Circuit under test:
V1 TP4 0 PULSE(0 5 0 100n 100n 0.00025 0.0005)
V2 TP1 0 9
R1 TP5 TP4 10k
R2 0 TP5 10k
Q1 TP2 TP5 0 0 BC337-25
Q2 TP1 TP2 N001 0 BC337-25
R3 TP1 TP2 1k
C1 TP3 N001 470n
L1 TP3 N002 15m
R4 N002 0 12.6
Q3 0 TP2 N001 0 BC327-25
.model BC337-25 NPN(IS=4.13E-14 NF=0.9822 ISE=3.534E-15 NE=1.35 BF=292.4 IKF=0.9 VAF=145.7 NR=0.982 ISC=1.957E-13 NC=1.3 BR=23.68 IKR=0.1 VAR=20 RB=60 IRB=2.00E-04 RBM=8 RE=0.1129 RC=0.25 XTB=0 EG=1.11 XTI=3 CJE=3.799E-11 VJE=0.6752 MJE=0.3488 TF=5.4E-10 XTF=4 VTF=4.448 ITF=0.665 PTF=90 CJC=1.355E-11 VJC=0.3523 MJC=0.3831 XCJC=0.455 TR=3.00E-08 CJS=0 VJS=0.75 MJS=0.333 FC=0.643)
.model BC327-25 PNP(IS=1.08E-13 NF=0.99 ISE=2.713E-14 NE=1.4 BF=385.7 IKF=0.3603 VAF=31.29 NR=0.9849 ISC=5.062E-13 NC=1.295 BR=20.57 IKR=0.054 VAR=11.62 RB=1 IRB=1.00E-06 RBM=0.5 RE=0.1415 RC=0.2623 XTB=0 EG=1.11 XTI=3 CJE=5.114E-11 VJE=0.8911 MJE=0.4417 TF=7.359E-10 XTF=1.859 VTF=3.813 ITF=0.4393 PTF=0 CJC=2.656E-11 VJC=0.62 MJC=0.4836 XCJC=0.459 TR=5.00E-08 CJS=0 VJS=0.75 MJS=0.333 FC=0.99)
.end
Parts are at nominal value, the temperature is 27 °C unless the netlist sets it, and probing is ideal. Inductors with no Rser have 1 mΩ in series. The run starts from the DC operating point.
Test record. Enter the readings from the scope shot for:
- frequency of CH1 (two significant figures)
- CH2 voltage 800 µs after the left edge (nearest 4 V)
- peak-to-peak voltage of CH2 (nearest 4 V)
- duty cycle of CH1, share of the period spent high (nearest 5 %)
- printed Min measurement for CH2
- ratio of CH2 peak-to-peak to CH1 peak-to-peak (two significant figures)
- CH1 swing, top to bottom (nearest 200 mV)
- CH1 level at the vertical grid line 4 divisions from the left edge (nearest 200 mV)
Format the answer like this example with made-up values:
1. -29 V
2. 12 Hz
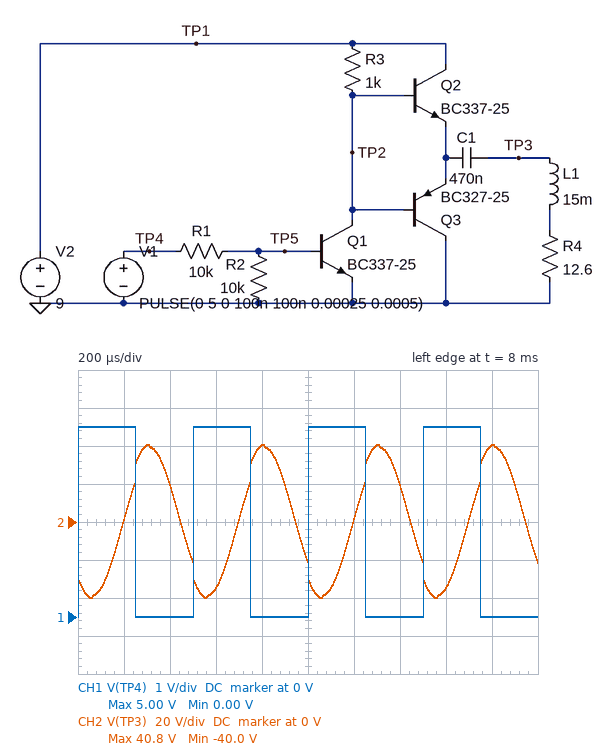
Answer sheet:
1. 2.0 kHz
2. 40 V
3. 80 V
4. 50 %
5. -40.0 V
6. 16
7. 5.0 V
8. 0 V
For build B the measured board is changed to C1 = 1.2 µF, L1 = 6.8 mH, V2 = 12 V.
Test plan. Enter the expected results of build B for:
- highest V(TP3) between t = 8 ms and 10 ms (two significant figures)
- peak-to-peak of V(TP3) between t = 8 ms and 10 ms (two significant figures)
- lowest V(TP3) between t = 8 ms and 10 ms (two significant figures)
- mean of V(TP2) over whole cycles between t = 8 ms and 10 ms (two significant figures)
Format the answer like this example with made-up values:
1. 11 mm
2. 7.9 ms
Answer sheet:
1. 26 V
2. 51 V
3. -25 V
4. 5.7 V
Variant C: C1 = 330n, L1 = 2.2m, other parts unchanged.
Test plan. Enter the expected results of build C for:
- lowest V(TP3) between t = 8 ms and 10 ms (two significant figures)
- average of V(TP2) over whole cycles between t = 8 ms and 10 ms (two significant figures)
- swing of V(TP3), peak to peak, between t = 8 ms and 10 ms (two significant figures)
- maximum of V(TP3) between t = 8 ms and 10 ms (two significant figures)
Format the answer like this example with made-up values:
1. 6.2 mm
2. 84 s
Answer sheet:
1. -11 V
2. 4.5 V
3. 23 V
4. 12 V
